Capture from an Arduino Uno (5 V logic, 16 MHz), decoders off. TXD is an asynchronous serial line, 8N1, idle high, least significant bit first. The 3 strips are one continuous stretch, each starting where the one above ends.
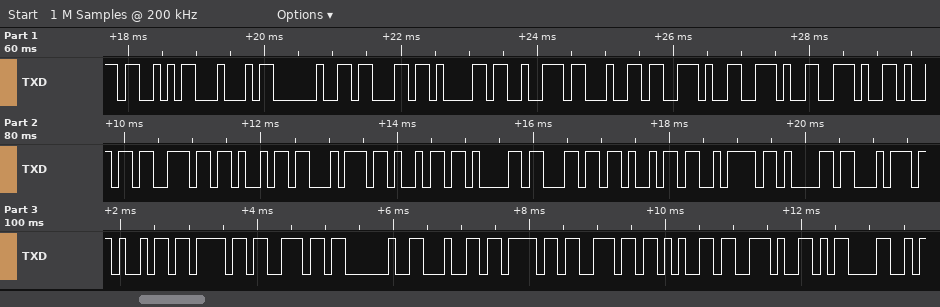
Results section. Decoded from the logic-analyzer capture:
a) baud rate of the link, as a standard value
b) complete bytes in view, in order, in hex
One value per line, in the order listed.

9600 baud
53 44 20 63 61 72 64 2E 2E 2E 69 6E 69 74 69 61 6C 69 7A 61 74 69 6F 6E 20 64 6F 6E 65 2E 0D
